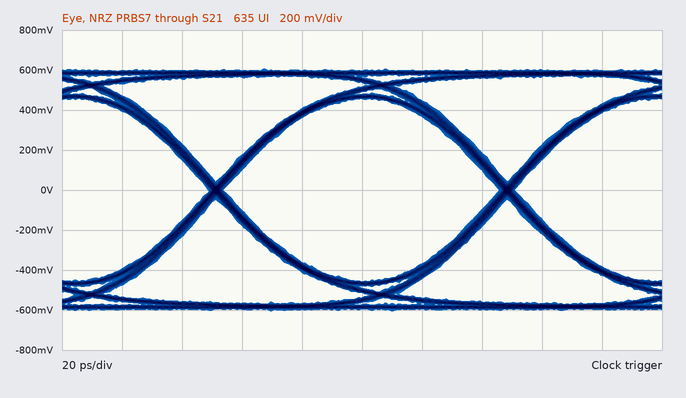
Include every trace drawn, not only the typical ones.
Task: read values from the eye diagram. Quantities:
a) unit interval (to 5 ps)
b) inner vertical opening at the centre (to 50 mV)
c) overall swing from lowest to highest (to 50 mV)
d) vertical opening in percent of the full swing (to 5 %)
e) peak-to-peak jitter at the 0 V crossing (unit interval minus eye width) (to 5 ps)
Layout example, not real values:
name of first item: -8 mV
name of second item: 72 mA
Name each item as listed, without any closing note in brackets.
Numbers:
unit interval: 95 ps
inner vertical opening at the centre: 900 mV
overall swing from lowest to highest: 1.20 V
vertical opening in percent of the full swing: 75 %
peak-to-peak jitter at the 0 V crossing (unit interval minus eye width): 5 ps
